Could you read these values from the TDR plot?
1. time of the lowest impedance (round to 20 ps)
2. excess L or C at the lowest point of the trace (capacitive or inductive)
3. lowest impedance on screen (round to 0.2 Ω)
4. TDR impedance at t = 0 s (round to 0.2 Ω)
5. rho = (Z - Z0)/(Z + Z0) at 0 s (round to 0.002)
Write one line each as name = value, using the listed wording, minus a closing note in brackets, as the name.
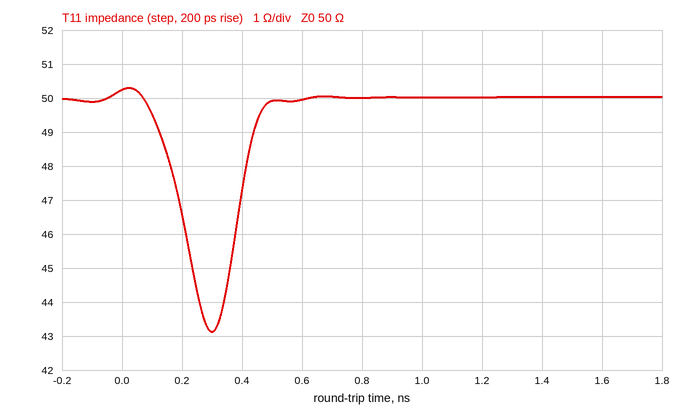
time of the lowest impedance = 300 ps
excess L or C at the lowest point of the trace = capacitive
lowest impedance on screen = 43.2 Ω
TDR impedance at t = 0 s = 50.2 Ω
rho = (Z - Z0)/(Z + Z0) at 0 s = +0.002
